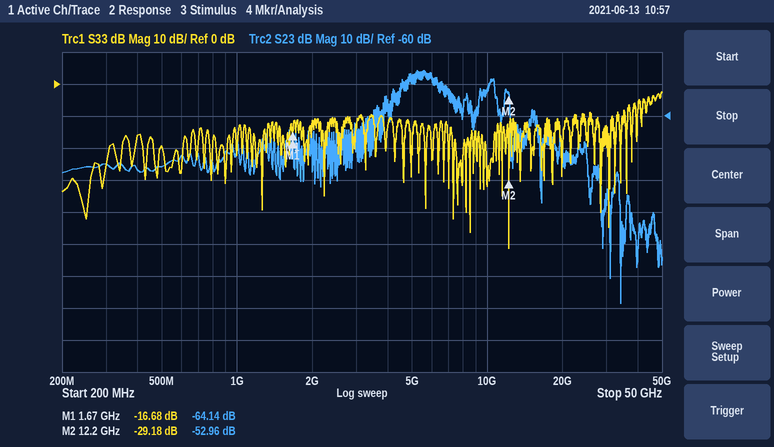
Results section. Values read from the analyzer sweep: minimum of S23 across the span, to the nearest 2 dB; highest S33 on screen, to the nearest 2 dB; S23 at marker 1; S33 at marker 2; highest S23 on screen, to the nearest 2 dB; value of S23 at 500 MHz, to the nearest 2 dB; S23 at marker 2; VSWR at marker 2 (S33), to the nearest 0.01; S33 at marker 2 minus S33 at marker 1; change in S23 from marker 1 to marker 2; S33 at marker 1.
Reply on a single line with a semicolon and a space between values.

-118 dB; -2 dB; -64.14 dB; -29.18 dB; -46 dB; -76 dB; -52.96 dB; 1.07; -12.50 dB; 11.18 dB; -16.68 dB
